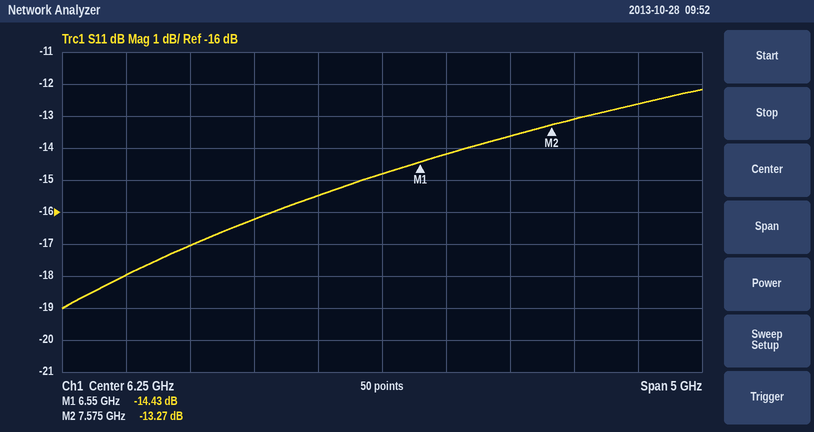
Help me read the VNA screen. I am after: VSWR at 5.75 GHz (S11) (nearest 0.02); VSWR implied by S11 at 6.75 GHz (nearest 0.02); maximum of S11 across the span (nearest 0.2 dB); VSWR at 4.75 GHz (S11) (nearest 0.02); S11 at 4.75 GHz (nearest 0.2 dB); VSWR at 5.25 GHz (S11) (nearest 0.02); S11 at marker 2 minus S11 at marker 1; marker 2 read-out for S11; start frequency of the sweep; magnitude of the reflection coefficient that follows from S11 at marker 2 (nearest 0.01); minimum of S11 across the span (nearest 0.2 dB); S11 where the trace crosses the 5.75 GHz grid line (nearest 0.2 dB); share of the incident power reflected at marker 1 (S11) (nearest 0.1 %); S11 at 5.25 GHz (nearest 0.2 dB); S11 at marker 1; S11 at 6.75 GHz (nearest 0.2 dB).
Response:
1.40
1.48
-12.2 dB
1.32
-17.0 dB
1.36
1.16 dB
-13.27 dB
3.75 GHz
0.22
-19.0 dB
-15.4 dB
3.6 %
-16.2 dB
-14.43 dB
-14.2 dB
